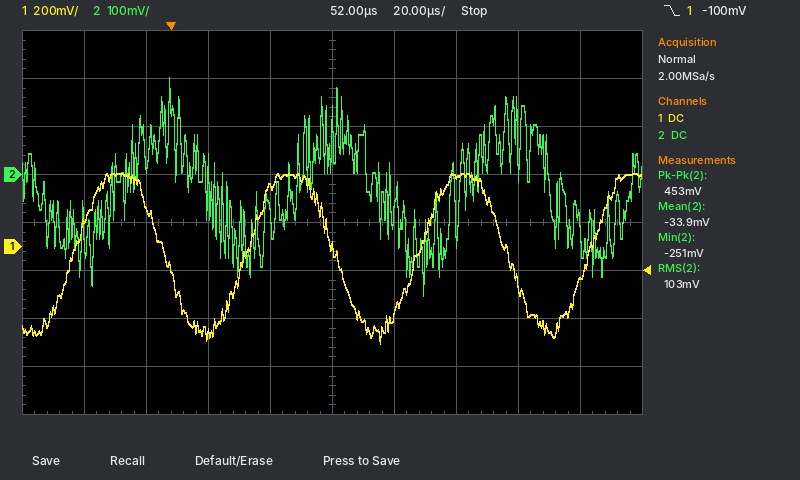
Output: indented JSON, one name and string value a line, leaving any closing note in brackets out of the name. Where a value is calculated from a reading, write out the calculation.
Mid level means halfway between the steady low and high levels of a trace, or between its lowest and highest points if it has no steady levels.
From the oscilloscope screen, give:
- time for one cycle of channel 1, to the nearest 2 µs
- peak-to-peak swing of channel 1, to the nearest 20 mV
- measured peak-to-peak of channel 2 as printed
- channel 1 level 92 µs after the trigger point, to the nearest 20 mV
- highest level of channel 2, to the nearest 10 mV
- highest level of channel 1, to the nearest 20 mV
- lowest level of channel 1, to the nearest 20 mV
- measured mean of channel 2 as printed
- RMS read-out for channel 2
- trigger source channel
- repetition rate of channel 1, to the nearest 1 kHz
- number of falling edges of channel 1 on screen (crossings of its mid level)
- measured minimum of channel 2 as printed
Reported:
{
  "time for one cycle of channel 1, to the nearest 2 µs": "56 µs",
  "peak-to-peak swing of channel 1, to the nearest 20 mV": "300 mV − (-400 mV) = 700 mV",
  "measured peak-to-peak of channel 2 as printed": "453 mV",
  "channel 1 level 92 µs after the trigger point, to the nearest 20 mV": "300 mV",
  "highest level of channel 2, to the nearest 10 mV": "200 mV",
  "highest level of channel 1, to the nearest 20 mV": "300 mV",
  "lowest level of channel 1, to the nearest 20 mV": "-400 mV",
  "measured mean of channel 2 as printed": "-33.9 mV",
  "RMS read-out for channel 2": "103 mV",
  "trigger source channel": "channel 1",
  "repetition rate of channel 1, to the nearest 1 kHz": "1 / 56 µs ≈ 18 kHz",
  "number of falling edges of channel 1 on screen": "3",
  "measured minimum of channel 2 as printed": "-251 mV"
}
